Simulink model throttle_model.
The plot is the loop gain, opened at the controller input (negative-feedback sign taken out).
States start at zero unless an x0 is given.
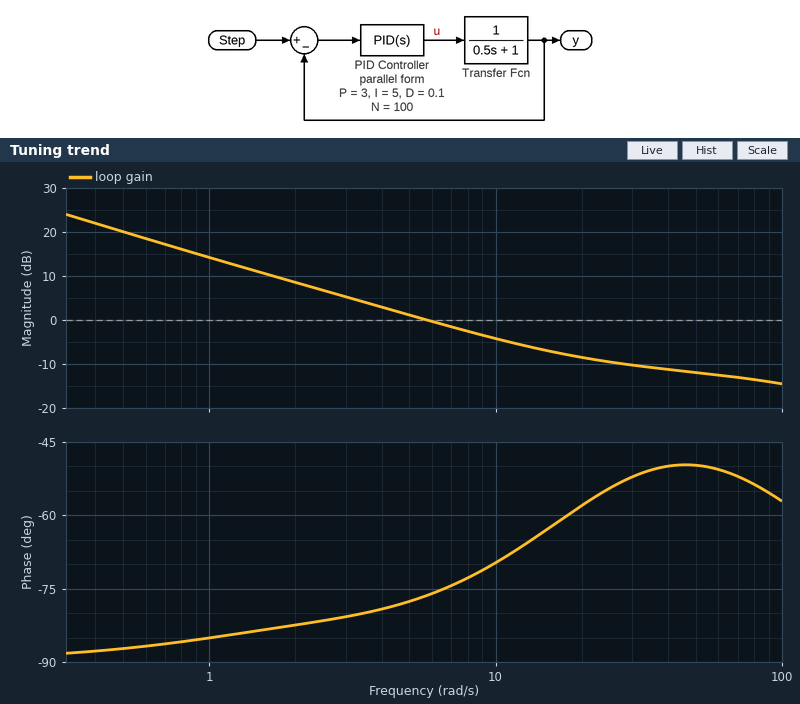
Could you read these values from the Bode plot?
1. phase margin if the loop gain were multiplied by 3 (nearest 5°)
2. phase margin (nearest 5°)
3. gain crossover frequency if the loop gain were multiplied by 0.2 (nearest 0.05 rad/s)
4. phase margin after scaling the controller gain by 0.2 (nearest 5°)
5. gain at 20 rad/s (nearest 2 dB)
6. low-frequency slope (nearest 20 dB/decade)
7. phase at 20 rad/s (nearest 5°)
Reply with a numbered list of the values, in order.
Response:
1. 125°
2. 105°
3. 1.05 rad/s
4. 95°
5. -8 dB
6. -20 dB/decade
7. -60°
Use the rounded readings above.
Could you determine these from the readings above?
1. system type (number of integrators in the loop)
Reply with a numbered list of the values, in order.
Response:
1. 1
